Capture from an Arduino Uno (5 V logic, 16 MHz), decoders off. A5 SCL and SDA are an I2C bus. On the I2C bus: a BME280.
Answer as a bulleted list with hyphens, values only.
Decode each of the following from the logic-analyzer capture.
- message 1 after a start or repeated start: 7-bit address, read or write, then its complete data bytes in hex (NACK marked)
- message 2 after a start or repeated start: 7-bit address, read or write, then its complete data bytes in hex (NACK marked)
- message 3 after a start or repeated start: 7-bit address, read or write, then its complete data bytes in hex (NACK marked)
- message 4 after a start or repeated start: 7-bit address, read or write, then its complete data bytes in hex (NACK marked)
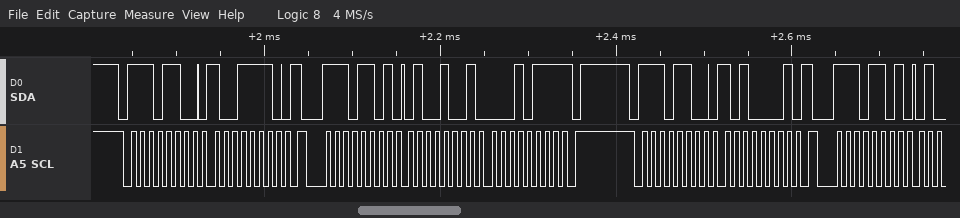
- 0x76 write: 9E
- 0x76 read: 49 17 NACK
- 0x76 write: A1
- 0x76 read
